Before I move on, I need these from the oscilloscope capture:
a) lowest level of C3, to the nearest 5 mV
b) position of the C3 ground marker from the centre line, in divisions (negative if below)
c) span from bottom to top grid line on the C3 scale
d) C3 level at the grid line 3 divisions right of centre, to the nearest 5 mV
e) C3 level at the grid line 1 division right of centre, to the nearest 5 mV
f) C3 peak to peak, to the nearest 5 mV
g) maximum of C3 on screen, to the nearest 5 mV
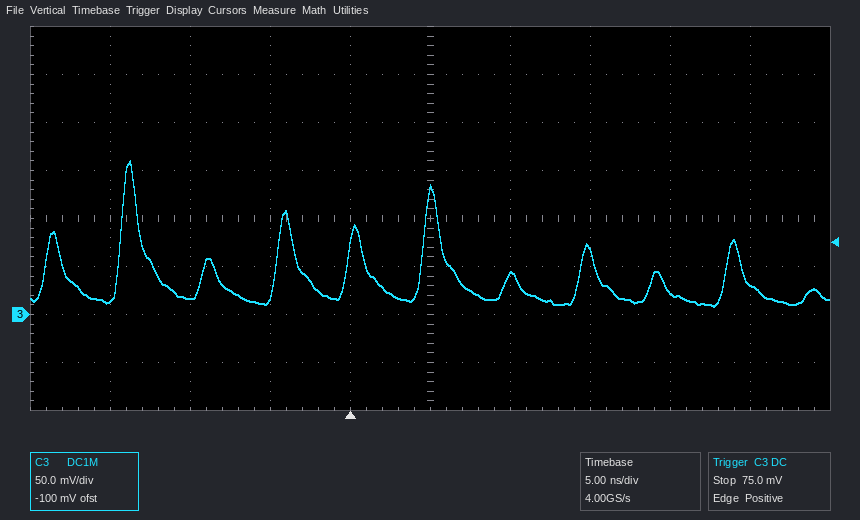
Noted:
10 mV
-2.0 div
400 mV
25 mV
40 mV
150 mV
160 mV
